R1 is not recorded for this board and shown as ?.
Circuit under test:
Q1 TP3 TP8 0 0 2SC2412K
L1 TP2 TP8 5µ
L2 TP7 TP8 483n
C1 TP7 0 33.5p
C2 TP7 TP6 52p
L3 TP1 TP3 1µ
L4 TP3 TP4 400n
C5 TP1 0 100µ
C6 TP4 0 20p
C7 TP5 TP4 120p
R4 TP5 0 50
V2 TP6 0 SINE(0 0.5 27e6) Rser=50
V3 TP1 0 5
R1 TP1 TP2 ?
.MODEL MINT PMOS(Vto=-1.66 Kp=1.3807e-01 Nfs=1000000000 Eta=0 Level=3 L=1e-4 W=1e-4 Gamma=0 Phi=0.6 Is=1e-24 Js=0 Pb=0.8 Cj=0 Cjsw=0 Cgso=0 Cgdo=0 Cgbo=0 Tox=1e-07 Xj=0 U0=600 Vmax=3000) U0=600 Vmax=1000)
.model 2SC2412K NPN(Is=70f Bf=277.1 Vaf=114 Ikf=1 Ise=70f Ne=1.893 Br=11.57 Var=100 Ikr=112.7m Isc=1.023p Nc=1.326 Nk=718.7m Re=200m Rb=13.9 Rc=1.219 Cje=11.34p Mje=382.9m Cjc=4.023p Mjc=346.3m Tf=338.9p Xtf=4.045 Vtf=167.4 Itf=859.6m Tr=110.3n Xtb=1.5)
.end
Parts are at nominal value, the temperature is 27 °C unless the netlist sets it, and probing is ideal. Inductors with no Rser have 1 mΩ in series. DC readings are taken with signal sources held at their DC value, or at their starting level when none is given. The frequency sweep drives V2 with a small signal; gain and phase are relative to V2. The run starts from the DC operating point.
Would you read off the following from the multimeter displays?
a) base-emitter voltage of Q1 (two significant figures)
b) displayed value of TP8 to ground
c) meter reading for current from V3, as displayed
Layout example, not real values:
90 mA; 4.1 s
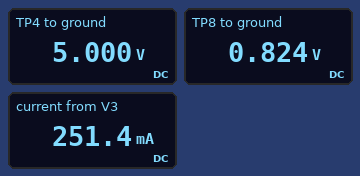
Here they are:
820 mV; 0.824 V; 251.4 mA
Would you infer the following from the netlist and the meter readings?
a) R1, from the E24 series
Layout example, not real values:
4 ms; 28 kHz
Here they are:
3.3 kΩ
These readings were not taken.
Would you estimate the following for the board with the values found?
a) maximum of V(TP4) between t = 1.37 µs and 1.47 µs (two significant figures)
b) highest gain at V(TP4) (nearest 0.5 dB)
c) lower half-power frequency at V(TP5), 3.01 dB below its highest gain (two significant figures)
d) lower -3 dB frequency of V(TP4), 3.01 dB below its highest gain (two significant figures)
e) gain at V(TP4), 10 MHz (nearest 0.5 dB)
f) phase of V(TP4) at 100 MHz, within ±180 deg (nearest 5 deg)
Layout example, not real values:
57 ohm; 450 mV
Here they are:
8.9 V; 21.5 dB; 11 MHz; 8.9 MHz; 20.5 dB; -105 deg
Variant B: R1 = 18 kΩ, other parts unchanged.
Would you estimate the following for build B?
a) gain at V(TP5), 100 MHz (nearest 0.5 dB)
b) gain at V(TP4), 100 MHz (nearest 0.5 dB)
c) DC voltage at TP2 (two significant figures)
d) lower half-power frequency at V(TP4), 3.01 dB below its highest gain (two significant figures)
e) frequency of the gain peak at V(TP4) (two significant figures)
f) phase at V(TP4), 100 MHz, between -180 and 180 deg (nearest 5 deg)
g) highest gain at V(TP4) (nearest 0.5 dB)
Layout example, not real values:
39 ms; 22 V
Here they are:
-15.5 dB; -15.0 dB; 730 mV; 8.6 MHz; 11 MHz; -115 deg; 25.0 dB
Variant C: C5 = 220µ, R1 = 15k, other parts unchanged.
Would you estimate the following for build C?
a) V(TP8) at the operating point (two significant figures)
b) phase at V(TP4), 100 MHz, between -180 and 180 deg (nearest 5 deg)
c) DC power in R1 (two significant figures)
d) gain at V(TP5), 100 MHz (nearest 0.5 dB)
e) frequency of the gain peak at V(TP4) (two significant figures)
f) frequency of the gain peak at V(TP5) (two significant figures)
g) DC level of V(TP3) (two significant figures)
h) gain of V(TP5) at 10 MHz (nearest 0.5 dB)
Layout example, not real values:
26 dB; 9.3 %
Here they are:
740 mV; -115 deg; 1.2 mW; -15.5 dB; 11 MHz; 25 MHz; 5.0 V; 15.5 dB
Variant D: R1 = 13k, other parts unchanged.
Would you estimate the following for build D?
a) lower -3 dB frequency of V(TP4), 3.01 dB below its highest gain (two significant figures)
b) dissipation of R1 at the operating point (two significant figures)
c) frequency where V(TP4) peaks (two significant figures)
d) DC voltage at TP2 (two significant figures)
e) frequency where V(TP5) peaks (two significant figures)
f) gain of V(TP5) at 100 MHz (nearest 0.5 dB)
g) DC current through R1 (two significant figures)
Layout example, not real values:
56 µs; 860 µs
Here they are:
8.6 MHz; 1.4 mW; 11 MHz; 740 mV; 25 MHz; -15.5 dB; 330 µA
